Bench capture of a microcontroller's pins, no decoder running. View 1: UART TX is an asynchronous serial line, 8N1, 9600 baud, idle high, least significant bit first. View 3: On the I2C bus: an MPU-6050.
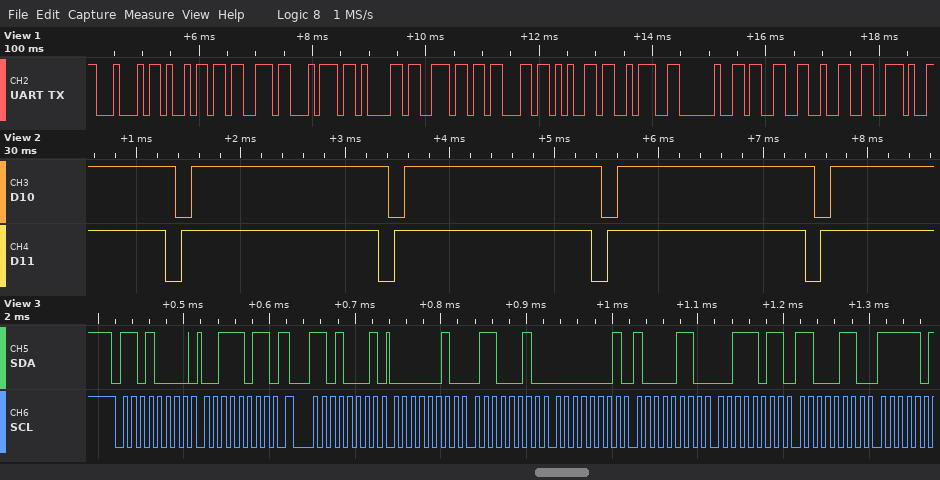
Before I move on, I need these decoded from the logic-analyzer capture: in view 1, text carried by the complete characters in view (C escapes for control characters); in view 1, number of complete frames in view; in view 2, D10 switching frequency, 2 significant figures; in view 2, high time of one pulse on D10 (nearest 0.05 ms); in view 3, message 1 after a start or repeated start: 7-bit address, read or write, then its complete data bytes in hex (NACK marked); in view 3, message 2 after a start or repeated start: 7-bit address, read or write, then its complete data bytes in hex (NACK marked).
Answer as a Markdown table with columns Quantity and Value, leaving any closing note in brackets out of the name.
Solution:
| Quantity | Value |
|---|---|
| in view 1, text carried by the complete characters in view | "Distance: 32." |
| in view 1, number of complete frames in view | 13 |
| in view 2, D10 switching frequency, 2 significant figures | 490 Hz |
| in view 2, high time of one pulse on D10 | 1.90 ms |
| in view 3, message 1 after a start or repeated start: 7-bit address, read or write, then its complete data bytes in hex | 0x68 write: 3B |
| in view 3, message 2 after a start or repeated start: 7-bit address, read or write, then its complete data bytes in hex | 0x68 read: 02 62 01 86 3B C6 |
